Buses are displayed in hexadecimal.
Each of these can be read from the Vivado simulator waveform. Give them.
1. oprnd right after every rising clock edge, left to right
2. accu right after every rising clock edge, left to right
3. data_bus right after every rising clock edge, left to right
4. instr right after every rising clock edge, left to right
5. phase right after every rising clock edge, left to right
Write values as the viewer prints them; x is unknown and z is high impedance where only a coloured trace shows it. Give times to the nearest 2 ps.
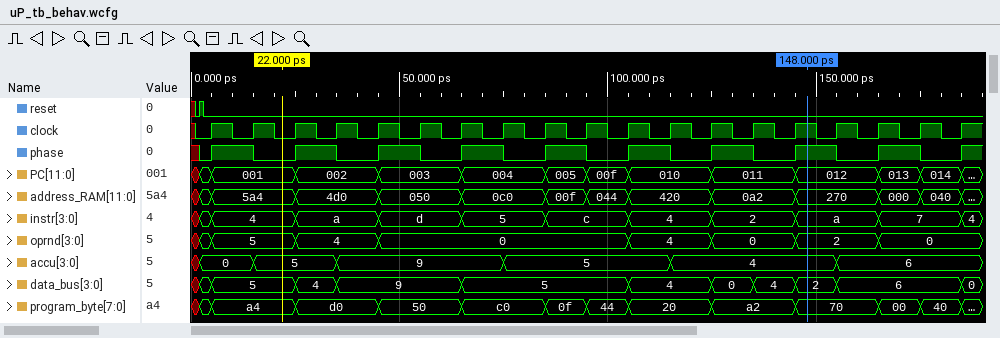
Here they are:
5, 5, 4, 4, 0, 0, 0, 0, 0, 0, 4, 4, 0, 0, 2, 2, 0, 0, 0
0, 5, 5, 9, 9, 9, 9, 5, 5, 5, 5, 4, 4, 4, 4, 6, 6, 6, 6
5, 5, 4, 9, 9, 9, 5, 5, 5, 5, 4, 4, 0, 4, 2, 6, 6, 6, 0
4, 4, a, a, d, d, 5, 5, c, c, 4, 4, 2, 2, a, a, 7, 7, 4
1 0 1 0 1 0 1 0 1 0 1 0 1 0 1 0 1 0 1
